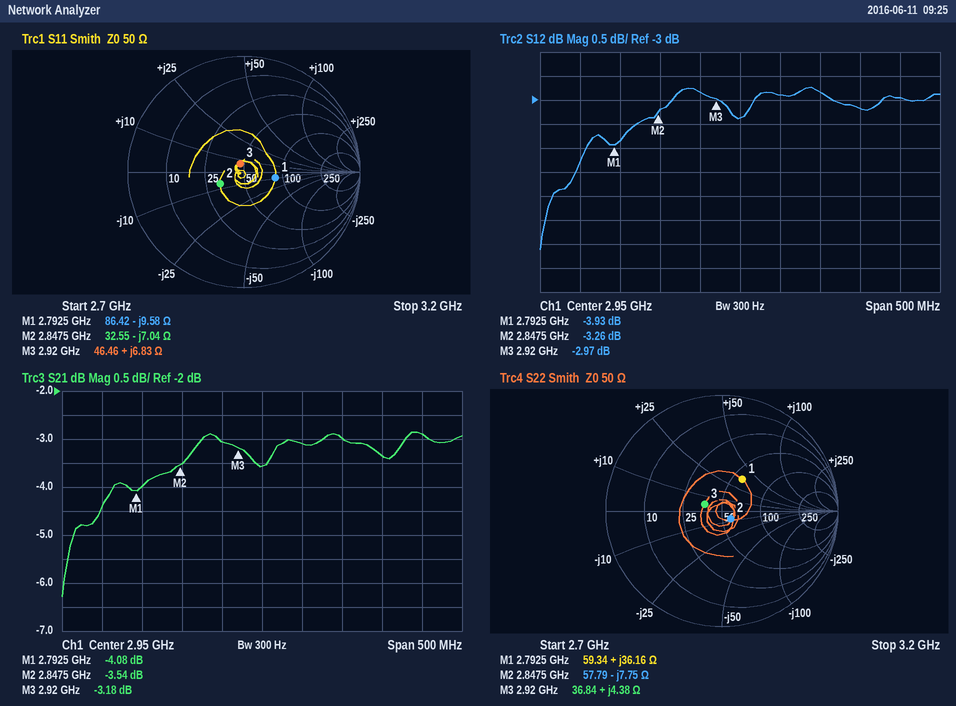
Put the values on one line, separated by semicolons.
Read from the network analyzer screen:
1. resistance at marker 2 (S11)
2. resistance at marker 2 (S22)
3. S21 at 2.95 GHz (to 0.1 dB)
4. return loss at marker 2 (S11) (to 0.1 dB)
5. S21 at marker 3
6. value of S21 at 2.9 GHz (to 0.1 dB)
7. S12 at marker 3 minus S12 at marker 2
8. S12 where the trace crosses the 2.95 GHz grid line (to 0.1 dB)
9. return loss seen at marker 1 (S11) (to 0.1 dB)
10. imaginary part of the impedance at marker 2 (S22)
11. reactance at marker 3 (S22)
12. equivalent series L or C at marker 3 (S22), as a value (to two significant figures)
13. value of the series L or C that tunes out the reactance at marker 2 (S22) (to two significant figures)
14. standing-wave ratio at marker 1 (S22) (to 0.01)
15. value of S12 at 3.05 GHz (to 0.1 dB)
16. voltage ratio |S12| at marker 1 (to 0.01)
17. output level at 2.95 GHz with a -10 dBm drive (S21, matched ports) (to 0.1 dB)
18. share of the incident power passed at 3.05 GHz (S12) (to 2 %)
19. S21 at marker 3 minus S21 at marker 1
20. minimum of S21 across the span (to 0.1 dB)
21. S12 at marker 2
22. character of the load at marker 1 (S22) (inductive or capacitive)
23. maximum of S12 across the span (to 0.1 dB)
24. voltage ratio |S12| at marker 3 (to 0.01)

32.55 Ω; 57.79 Ω; -3.6 dB; 12.9 dB; -3.18 dB; -3.1 dB; 0.29 dB; -3.4 dB; 11.2 dB; -7.75 Ω; +4.38 Ω; 240 pH; 430 pH; 1.96; -2.8 dB; 0.64; -13.6 dBm; 52 %; 0.90 dB; -6.3 dB; -3.26 dB; inductive; -2.7 dB; 0.71
